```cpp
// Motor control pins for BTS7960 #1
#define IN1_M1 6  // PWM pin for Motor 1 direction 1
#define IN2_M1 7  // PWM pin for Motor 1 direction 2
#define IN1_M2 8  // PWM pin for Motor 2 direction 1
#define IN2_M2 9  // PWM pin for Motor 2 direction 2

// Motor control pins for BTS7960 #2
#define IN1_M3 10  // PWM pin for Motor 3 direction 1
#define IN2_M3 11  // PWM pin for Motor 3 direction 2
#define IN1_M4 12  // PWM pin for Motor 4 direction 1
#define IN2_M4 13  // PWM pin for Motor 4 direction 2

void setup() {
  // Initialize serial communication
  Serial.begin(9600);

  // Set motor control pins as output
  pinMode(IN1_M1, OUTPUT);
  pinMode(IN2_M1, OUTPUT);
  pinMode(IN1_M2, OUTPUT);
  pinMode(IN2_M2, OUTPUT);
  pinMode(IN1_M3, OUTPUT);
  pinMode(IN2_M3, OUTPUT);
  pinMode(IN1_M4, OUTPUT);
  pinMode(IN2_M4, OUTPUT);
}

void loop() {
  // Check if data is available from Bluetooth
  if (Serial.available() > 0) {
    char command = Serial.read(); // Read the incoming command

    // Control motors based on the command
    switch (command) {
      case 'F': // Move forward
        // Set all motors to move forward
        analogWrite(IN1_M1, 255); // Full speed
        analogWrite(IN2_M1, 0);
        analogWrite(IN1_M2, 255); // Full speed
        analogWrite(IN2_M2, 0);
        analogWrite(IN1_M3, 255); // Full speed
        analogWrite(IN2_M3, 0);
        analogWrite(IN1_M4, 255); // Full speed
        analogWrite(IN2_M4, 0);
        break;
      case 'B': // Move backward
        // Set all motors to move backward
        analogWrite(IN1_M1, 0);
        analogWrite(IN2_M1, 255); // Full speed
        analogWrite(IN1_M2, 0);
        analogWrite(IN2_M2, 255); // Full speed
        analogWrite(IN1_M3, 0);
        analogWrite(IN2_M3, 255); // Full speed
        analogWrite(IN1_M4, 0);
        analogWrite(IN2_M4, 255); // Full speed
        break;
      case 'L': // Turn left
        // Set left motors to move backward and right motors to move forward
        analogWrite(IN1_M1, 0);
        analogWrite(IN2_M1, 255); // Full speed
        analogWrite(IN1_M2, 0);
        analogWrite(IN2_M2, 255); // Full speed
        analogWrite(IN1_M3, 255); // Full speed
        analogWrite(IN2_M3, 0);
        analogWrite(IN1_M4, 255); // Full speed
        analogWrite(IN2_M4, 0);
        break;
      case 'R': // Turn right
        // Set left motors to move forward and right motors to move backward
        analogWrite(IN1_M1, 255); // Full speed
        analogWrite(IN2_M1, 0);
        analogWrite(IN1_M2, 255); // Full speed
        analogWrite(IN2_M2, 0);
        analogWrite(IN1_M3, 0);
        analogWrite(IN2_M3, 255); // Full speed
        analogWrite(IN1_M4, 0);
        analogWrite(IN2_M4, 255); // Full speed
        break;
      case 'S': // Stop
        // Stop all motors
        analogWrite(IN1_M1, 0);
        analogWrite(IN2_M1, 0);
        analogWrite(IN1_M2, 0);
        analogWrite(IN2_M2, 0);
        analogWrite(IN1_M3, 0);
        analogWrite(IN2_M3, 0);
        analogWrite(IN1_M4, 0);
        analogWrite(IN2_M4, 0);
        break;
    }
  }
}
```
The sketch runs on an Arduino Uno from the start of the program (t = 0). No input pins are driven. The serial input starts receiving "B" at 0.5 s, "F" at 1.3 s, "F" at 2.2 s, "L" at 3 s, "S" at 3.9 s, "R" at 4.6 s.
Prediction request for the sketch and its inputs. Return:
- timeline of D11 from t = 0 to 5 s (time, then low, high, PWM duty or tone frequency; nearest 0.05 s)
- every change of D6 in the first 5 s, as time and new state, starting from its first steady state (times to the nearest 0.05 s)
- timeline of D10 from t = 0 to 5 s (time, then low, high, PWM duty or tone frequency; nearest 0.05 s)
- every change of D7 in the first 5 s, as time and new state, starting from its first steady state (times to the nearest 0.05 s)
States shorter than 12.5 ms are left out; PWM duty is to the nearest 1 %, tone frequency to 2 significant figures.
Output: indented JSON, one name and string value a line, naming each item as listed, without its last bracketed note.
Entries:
{
  "timeline of D11 from t = 0 to 5 s": "0 s low; 0.5 s high; 1.3 s low; 4.6 s high",
  "every change of D6 in the first 5 s, as time and new state, starting from its first steady state": "0 s low; 1.3 s high; 3 s low; 4.6 s high",
  "timeline of D10 from t = 0 to 5 s": "0 s low; 1.3 s high; 3.9 s low",
  "every change of D7 in the first 5 s, as time and new state, starting from its first steady state": "0 s low; 0.5 s high; 1.3 s low; 3 s high; 3.9 s low"
}
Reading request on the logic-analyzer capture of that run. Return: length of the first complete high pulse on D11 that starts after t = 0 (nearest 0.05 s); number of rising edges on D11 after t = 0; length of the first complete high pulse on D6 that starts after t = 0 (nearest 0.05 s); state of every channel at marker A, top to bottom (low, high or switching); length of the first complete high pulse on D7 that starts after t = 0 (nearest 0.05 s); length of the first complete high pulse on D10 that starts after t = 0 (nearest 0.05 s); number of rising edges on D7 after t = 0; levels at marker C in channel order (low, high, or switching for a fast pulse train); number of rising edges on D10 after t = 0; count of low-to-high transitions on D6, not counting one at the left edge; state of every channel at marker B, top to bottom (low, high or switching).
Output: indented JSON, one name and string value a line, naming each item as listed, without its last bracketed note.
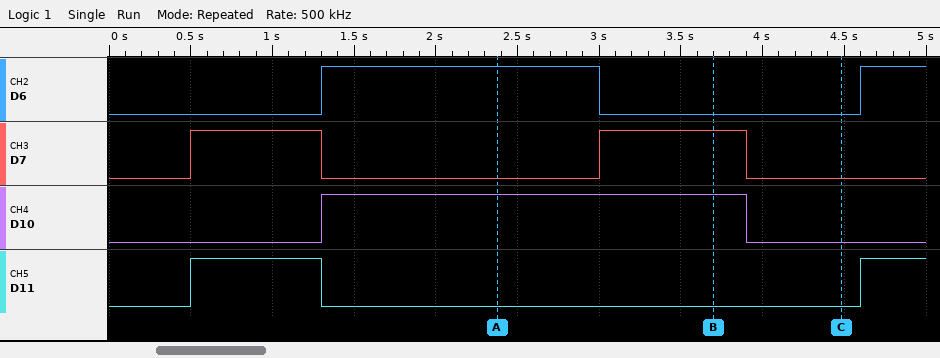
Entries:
{
  "length of the first complete high pulse on D11 that starts after t = 0": "0.80 s",
  "number of rising edges on D11 after t = 0": "2",
  "length of the first complete high pulse on D6 that starts after t = 0": "1.70 s",
  "state of every channel at marker A, top to bottom": "D6 high, D7 low, D10 high, D11 low",
  "length of the first complete high pulse on D7 that starts after t = 0": "0.80 s",
  "length of the first complete high pulse on D10 that starts after t = 0": "2.60 s",
  "number of rising edges on D7 after t = 0": "2",
  "levels at marker C in channel order": "D6 low, D7 low, D10 low, D11 low",
  "number of rising edges on D10 after t = 0": "1",
  "count of low-to-high transitions on D6, not counting one at the left edge": "2",
  "state of every channel at marker B, top to bottom": "D6 low, D7 high, D10 high, D11 low"
}
